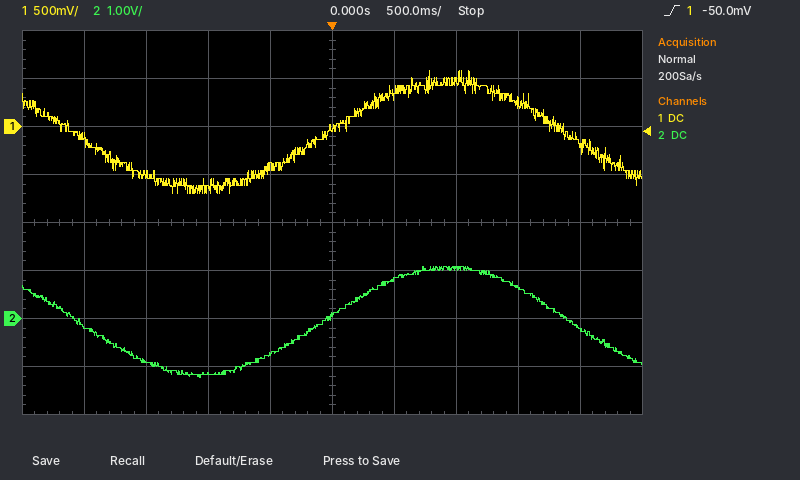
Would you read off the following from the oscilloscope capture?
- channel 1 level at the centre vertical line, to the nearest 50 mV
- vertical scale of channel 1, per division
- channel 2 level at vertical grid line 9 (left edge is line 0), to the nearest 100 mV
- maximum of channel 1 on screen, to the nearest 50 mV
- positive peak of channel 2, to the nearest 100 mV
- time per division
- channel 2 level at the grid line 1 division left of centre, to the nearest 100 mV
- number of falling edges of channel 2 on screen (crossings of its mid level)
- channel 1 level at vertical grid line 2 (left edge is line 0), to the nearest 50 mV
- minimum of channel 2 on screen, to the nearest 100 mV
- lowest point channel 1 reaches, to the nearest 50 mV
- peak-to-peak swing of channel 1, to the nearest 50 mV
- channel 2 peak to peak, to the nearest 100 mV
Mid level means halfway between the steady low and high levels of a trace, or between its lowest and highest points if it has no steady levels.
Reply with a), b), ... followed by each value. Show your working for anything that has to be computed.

a) 0 mV
b) 500 mV
c) -200 mV
d) 600 mV
e) 1.1 V
f) 500 ms
g) -700 mV
h) 2
i) -500 mV
j) -1.2 V
k) -700 mV
l) 600 mV − (-700 mV) = 1.30 V
m) 1.1 V − (-1.2 V) = 2.3 V
